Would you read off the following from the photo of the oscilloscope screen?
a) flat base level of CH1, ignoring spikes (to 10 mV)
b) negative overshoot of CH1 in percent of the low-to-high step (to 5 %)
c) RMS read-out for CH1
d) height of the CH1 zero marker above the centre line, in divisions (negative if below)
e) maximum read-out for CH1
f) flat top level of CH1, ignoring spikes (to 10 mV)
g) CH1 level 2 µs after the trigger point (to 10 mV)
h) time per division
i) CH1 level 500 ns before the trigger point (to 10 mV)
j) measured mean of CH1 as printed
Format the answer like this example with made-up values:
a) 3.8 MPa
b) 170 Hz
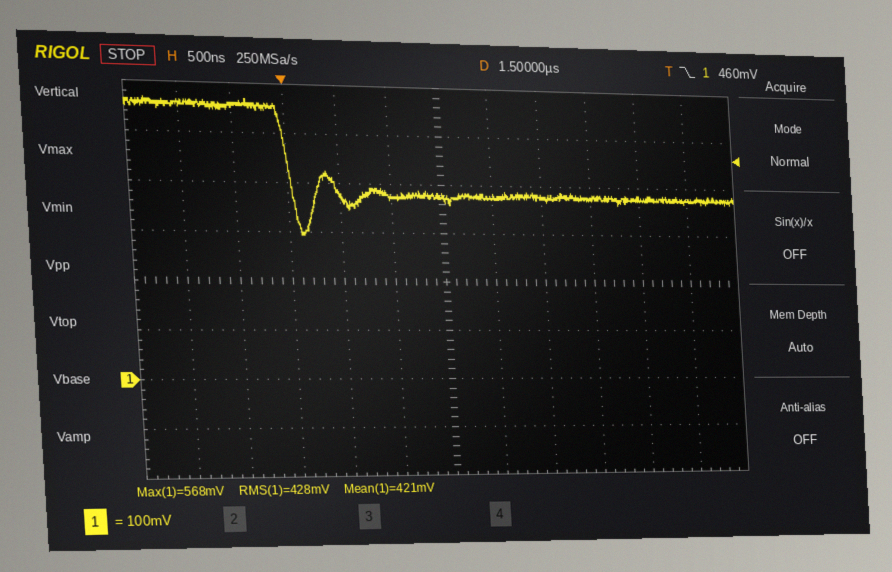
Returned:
a) 380 mV
b) 45 %
c) 428 mV
d) -2.0 div
e) 568 mV
f) 560 mV
g) 380 mV
h) 500 ns
i) 560 mV
j) 421 mV
